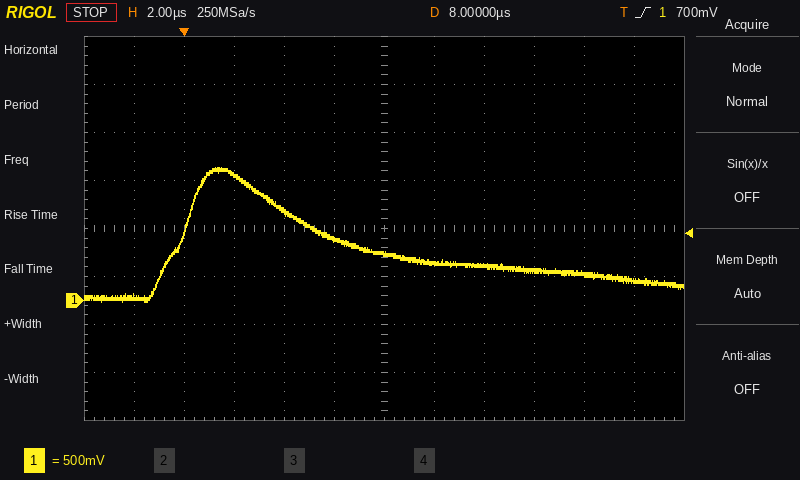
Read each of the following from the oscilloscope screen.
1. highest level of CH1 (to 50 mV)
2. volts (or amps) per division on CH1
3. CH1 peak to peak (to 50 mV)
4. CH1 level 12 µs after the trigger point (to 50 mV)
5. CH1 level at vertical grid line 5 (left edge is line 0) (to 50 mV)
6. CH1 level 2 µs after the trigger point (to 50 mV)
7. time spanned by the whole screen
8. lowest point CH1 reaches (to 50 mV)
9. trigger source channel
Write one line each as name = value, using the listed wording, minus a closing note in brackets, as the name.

highest level of CH1 = 1.40 V
volts (or amps) per division on CH1 = 500 mV
CH1 peak to peak = 1.40 V
CH1 level 12 µs after the trigger point = 350 mV
CH1 level at vertical grid line 5 (left edge is line 0) = 650 mV
CH1 level 2 µs after the trigger point = 1.30 V
time spanned by the whole screen = 24 µs
lowest point CH1 reaches = 0 mV
trigger source channel = CH1
